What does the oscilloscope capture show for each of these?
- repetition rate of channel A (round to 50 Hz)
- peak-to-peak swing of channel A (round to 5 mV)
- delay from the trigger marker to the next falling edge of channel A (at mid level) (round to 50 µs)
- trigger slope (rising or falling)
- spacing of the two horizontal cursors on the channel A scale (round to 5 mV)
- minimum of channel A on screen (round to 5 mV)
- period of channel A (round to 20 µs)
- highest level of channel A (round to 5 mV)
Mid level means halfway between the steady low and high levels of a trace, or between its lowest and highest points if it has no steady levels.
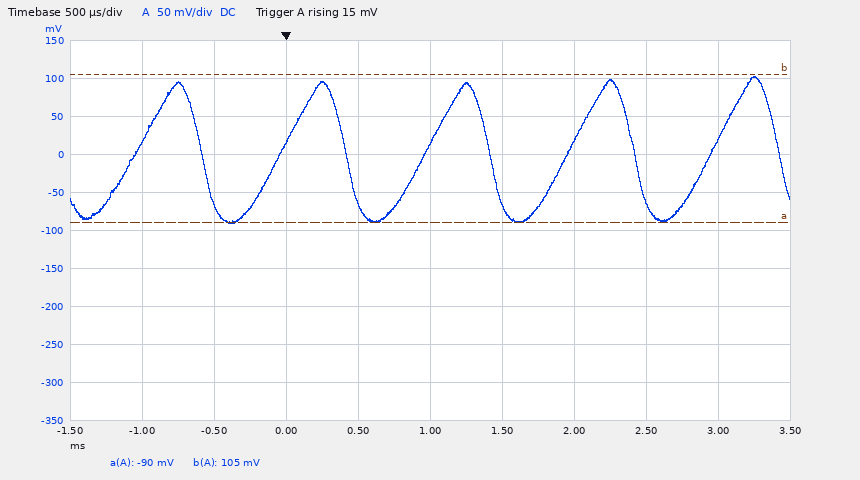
1.00 kHz
195 mV
400 µs
rising
195 mV
-90 mV
1.00 ms
105 mV
